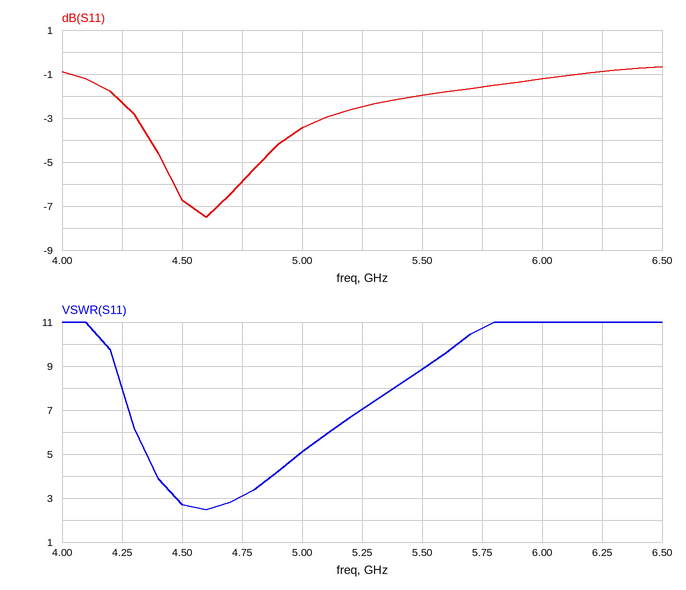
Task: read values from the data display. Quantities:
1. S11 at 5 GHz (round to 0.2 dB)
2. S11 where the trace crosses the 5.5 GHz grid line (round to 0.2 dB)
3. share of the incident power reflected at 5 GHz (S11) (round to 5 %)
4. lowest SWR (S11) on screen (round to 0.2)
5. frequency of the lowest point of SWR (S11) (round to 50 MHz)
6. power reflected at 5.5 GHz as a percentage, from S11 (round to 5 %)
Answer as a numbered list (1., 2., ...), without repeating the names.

1. -3.4 dB
2. -2.0 dB
3. 45 %
4. 2.4
5. 4.60 GHz
6. 65 %
